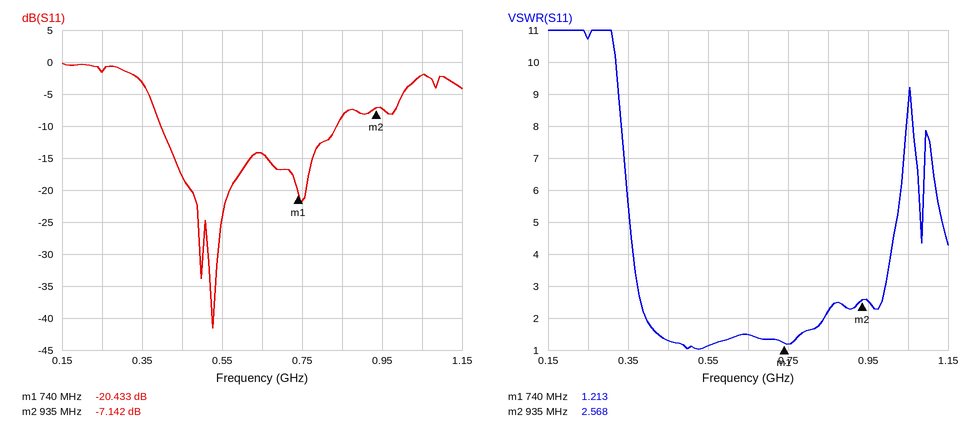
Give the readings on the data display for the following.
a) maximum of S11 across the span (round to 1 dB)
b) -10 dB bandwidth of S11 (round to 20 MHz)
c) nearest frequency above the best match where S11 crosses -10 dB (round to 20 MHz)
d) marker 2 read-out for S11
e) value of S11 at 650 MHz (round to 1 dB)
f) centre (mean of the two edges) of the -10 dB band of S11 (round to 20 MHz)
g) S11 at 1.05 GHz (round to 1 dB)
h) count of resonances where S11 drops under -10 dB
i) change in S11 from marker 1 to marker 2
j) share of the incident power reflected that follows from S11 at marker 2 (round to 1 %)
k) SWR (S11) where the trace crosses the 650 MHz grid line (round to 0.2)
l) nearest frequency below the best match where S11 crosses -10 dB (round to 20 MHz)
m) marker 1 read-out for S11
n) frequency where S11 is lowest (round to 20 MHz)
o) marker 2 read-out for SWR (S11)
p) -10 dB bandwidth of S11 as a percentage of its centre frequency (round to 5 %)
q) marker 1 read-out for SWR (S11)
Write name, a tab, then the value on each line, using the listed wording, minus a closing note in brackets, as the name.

maximum of S11 across the span	0 dB
-10 dB bandwidth of S11	440 MHz
nearest frequency above the best match where S11 crosses -10 dB	840 MHz
marker 2 read-out for S11	-7.142 dB
value of S11 at 650 MHz	-14 dB
centre (mean of the two edges) of the -10 dB band of S11	620 MHz
S11 at 1.05 GHz	-2 dB
count of resonances where S11 drops under -10 dB	3
change in S11 from marker 1 to marker 2	13.291 dB
share of the incident power reflected that follows from S11 at marker 2	19 %
SWR (S11) where the trace crosses the 650 MHz grid line	1.4
nearest frequency below the best match where S11 crosses -10 dB	400 MHz
marker 1 read-out for S11	-20.433 dB
frequency where S11 is lowest	520 MHz
marker 2 read-out for SWR	2.568
-10 dB bandwidth of S11 as a percentage of its centre frequency	70 %
marker 1 read-out for SWR	1.213
